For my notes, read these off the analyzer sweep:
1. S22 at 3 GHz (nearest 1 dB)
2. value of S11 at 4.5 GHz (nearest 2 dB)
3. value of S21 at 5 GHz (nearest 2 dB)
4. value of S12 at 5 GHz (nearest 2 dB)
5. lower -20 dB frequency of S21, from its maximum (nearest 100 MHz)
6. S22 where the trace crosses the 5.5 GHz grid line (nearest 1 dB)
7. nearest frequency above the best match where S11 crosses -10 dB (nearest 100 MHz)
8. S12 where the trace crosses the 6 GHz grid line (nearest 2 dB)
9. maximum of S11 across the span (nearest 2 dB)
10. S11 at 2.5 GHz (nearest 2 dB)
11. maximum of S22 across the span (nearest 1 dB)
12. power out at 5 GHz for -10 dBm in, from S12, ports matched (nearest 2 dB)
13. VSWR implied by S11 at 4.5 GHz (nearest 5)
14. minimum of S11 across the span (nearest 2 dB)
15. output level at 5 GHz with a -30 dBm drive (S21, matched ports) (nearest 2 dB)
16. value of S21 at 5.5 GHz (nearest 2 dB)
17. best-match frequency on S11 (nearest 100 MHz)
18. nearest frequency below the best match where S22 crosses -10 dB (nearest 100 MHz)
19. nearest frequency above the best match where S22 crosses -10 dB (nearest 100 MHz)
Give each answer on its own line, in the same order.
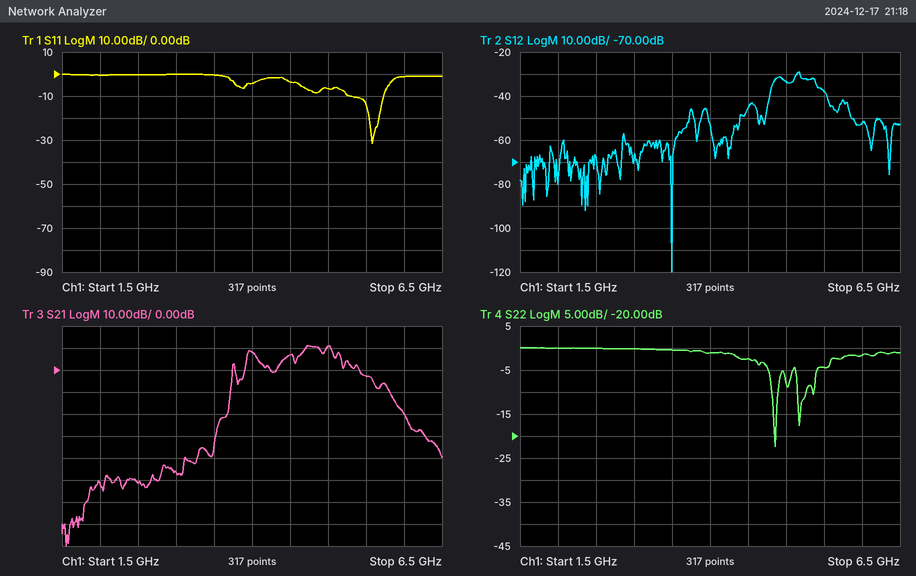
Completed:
0 dB
-4 dB
10 dB
-34 dB
3.7 GHz
-4 dB
5.7 GHz
-52 dB
0 dB
0 dB
0 dB
-44 dBm
5
-32 dB
-20 dBm
-2 dB
5.6 GHz
4.8 GHz
4.9 GHz
